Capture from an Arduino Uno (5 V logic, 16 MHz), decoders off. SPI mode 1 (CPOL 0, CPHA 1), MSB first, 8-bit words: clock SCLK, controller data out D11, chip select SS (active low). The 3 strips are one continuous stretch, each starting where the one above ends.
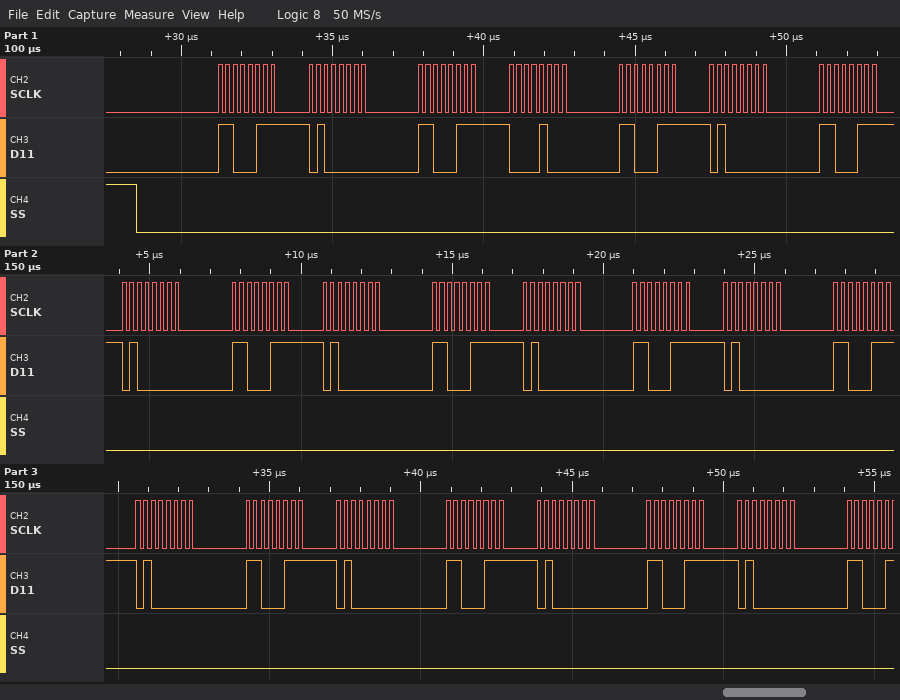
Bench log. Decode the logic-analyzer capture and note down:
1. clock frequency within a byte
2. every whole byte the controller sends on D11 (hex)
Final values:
4 MHz
C7 40 C7 08 C7 40 C7 40 C7 40 C7 40 C7 40 C7 40 C7 40 C7 40 C7 40
